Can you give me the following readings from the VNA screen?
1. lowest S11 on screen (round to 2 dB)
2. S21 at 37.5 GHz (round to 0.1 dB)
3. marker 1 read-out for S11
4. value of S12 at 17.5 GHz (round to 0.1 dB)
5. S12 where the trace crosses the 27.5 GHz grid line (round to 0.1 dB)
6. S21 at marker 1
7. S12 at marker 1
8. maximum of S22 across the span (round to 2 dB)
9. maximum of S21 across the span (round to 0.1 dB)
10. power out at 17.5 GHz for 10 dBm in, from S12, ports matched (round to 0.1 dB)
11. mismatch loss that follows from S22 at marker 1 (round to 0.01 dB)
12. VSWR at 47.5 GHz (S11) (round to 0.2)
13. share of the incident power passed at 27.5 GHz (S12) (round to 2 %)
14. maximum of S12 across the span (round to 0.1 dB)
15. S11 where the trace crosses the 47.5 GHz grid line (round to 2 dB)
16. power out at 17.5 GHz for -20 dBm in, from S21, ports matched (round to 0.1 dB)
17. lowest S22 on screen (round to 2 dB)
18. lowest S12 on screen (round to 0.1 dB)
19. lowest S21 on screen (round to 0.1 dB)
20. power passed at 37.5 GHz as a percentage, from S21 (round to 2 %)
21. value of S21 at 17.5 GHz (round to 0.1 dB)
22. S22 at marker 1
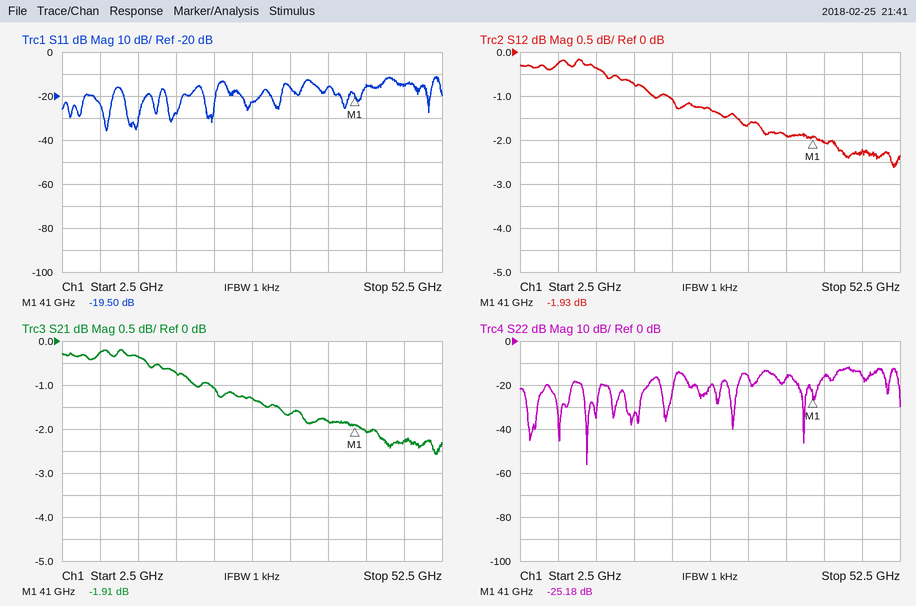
-36 dB
-1.8 dB
-19.50 dB
-0.7 dB
-1.3 dB
-1.91 dB
-1.93 dB
-12 dB
-0.2 dB
9.3 dBm
0.01 dB
1.4
74 %
-0.2 dB
-16 dB
-20.7 dBm
-56 dB
-2.6 dB
-2.6 dB
66 %
-0.7 dB
-25.18 dB
